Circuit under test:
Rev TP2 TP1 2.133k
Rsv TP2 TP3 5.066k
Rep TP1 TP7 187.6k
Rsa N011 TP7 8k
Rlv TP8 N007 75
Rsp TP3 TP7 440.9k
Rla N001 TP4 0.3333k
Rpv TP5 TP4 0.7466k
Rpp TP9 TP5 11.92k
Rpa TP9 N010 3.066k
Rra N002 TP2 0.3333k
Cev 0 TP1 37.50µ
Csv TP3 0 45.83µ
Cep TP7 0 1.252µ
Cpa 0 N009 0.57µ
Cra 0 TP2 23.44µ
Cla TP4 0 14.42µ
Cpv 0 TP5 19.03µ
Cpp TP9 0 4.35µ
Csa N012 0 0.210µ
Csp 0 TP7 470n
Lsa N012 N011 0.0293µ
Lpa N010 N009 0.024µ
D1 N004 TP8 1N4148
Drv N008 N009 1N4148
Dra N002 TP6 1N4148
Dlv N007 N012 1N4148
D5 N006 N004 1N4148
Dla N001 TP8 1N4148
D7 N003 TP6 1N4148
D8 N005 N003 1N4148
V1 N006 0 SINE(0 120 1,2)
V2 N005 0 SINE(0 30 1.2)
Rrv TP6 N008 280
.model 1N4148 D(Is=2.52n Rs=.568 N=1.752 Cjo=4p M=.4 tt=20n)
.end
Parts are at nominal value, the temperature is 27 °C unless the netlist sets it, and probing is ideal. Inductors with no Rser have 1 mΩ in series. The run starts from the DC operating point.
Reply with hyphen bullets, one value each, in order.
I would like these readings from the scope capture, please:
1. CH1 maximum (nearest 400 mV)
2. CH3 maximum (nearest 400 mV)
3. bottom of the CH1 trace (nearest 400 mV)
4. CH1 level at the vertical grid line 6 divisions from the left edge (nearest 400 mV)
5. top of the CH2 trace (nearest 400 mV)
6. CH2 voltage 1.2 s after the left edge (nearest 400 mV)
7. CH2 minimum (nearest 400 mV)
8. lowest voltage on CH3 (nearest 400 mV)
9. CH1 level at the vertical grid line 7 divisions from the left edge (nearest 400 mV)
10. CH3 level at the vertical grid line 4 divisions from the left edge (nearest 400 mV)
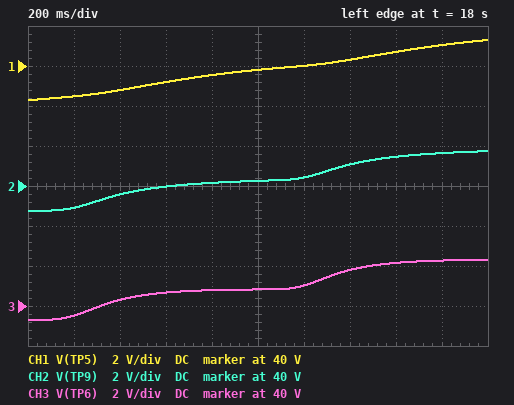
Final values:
- 41.2 V
- 42.4 V
- 38.4 V
- 40.0 V
- 41.6 V
- 40.4 V
- 38.8 V
- 39.2 V
- 40.4 V
- 40.8 V
